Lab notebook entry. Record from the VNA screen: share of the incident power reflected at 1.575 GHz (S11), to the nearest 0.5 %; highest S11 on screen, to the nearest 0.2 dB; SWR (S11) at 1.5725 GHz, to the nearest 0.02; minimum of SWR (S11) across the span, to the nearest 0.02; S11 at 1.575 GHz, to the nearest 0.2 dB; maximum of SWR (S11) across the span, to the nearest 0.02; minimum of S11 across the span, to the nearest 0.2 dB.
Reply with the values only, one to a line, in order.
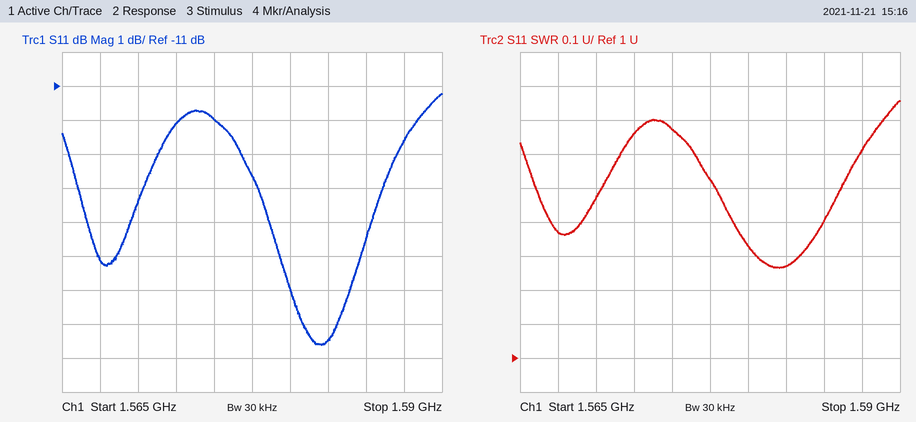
6.5 %
-11.2 dB
1.66
1.26
-12.0 dB
1.76
-18.6 dB
